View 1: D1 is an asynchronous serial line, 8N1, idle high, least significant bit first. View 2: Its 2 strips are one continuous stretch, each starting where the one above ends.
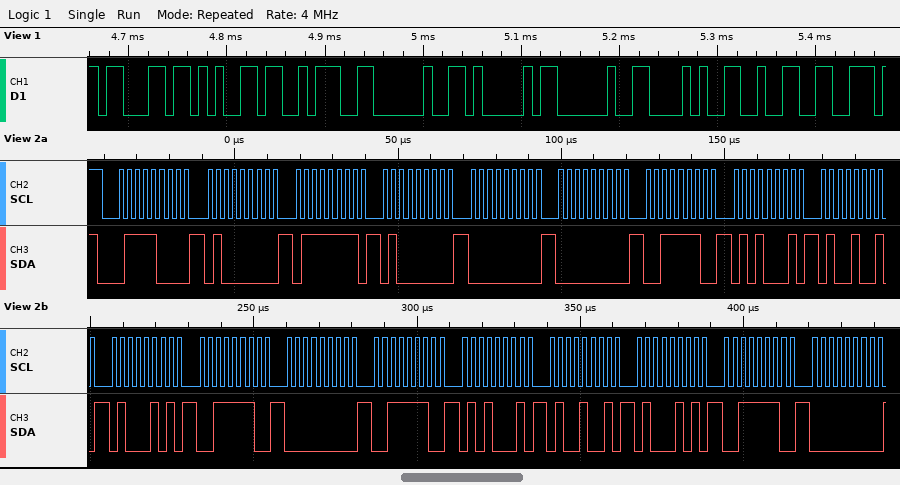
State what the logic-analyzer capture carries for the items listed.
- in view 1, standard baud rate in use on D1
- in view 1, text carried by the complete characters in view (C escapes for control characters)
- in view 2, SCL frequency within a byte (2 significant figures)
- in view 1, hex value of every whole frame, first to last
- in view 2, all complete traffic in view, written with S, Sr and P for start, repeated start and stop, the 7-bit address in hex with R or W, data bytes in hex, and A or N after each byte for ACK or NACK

115200 baud
"ce: A (2"
400 kHz
63 65 3A 20 41 20 28 32
S 3CW A 40 A 7F A 40 A 00 A 00 A 3E A 51 A 49 A 45 A 3E A 00 A 3E A 51 A 49 A 45 A 3E A 00 A
